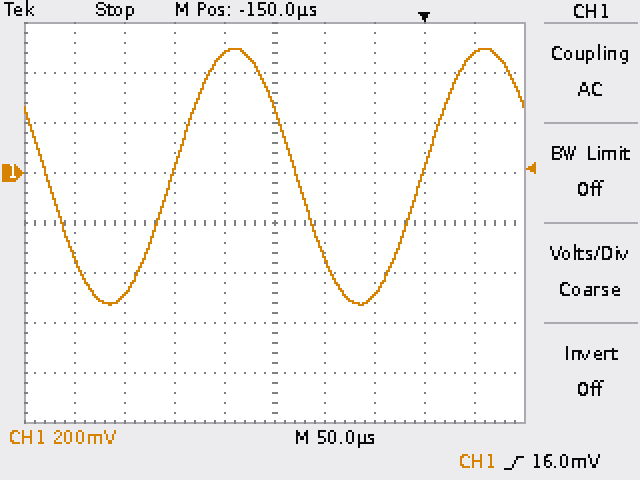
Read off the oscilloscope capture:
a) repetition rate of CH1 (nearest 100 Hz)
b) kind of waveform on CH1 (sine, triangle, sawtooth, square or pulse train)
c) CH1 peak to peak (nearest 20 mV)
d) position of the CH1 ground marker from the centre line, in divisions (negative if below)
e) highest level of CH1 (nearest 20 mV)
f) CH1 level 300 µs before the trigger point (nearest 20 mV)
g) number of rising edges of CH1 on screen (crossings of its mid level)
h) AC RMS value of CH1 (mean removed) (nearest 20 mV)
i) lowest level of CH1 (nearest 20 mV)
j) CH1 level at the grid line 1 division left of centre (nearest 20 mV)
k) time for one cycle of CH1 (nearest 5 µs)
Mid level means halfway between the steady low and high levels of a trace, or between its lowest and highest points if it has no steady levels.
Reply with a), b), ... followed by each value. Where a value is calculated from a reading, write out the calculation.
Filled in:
a) 1 / 250 µs ≈ 4.0 kHz
b) sine
c) 500 mV − (-520 mV) = 1.02 V
d) +1.0 div
e) 500 mV
f) -480 mV
g) 2
h) 1.02 V / (2√2) ≈ 361 mV, so 360 mV to the nearest 20 mV
i) -520 mV
j) 480 mV
k) 250 µs
